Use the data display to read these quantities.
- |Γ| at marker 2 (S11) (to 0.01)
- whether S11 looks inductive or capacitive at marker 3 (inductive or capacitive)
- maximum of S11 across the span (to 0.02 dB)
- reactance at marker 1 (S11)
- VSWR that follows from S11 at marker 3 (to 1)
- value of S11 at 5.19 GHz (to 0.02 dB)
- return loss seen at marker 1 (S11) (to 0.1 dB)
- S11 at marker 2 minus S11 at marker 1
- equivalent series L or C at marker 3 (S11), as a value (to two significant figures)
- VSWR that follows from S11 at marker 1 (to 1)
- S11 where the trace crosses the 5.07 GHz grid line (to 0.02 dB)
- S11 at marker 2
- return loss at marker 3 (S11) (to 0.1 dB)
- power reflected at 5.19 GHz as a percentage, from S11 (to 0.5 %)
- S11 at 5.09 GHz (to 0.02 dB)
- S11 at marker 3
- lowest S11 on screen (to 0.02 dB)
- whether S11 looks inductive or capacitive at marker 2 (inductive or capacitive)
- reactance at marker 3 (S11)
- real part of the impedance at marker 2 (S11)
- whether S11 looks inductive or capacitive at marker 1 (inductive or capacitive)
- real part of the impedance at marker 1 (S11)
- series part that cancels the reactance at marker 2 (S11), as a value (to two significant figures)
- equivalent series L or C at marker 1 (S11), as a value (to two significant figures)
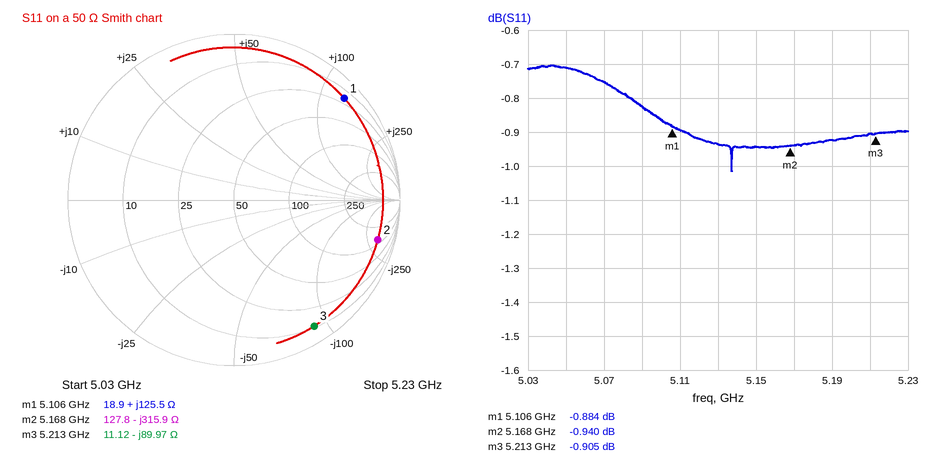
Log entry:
0.90
capacitive
-0.70 dB
+125.5 Ω
19
-0.92 dB
0.9 dB
-0.056 dB
340 fF
20
-0.76 dB
-0.940 dB
0.9 dB
81.0 %
-0.82 dB
-0.905 dB
-1.02 dB
capacitive
-89.97 Ω
127.8 Ω
inductive
18.9 Ω
9.7 nH
3.9 nH
